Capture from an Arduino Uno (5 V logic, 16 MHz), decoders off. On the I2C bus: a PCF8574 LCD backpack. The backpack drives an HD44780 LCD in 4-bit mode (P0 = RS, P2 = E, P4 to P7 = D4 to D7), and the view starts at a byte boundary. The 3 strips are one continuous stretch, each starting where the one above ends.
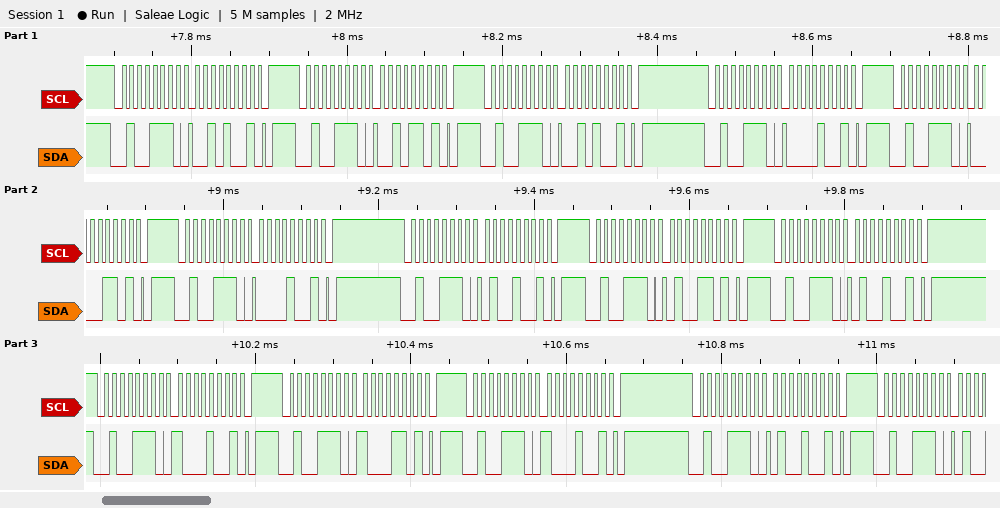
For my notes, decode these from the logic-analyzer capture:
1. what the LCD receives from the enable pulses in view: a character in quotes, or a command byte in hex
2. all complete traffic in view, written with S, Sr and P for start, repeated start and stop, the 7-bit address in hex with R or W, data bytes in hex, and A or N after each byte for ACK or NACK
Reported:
' ' 'H'
S 27W A 29 A P S 27W A 2D A P S 27W A 29 A P S 27W A 09 A P S 27W A 0D A P S 27W A 09 A P S 27W A 49 A P S 27W A 4D A P S 27W A 49 A P S 27W A 89 A P S 27W A 8D A P S 27W A 89 A P S 27W A 49 A P S 27W A
